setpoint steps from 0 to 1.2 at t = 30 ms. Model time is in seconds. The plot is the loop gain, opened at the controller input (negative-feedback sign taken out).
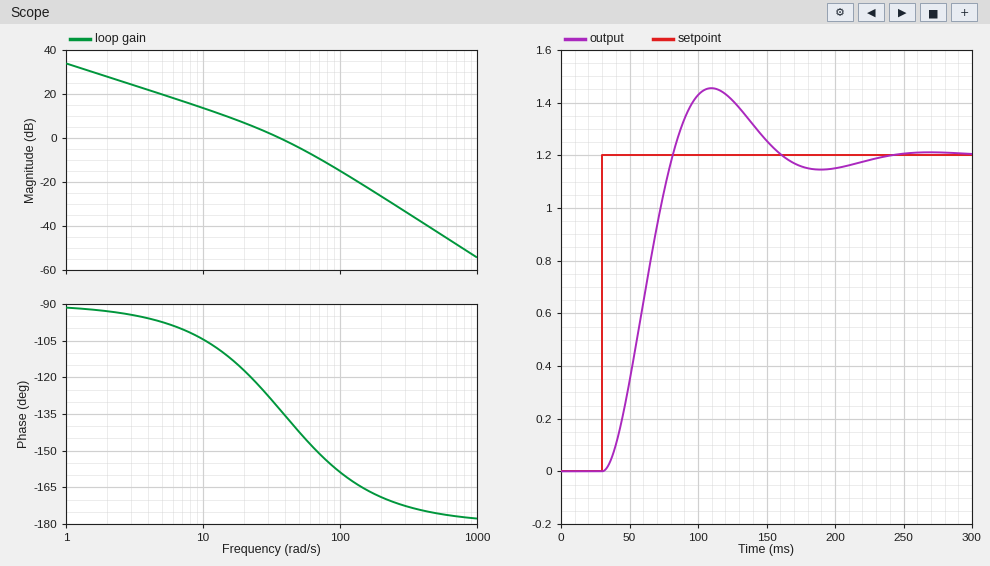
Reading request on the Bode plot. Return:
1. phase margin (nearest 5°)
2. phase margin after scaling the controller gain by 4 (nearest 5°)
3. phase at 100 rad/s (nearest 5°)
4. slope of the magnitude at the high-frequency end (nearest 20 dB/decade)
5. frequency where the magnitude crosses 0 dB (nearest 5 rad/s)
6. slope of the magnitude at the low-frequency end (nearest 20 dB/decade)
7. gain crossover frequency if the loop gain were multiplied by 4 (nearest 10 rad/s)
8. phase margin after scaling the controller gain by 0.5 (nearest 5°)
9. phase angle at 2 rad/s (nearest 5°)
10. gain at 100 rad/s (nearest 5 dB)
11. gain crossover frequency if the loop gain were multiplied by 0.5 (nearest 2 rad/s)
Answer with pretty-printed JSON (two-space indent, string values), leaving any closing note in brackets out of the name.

{
  "phase margin": "45°",
  "phase margin after scaling the controller gain by 4": "25°",
  "phase at 100 rad/s": "-160°",
  "slope of the magnitude at the high-frequency end": "-40 dB/decade",
  "frequency where the magnitude crosses 0 dB": "35 rad/s",
  "slope of the magnitude at the low-frequency end": "-20 dB/decade",
  "gain crossover frequency if the loop gain were multiplied by 4": "80 rad/s",
  "phase margin after scaling the controller gain by 0.5": "60°",
  "phase angle at 2 rad/s": "-95°",
  "gain at 100 rad/s": "-15 dB",
  "gain crossover frequency if the loop gain were multiplied by 0.5": "22 rad/s"
}
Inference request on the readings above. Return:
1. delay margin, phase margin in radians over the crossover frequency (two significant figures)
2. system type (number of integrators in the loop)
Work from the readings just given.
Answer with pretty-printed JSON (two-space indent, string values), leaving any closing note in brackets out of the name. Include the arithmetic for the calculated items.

{
  "delay margin, phase margin in radians over the crossover frequency": "45 × π / 180 / 35 = 0.022 s",
  "system type": "1"
}
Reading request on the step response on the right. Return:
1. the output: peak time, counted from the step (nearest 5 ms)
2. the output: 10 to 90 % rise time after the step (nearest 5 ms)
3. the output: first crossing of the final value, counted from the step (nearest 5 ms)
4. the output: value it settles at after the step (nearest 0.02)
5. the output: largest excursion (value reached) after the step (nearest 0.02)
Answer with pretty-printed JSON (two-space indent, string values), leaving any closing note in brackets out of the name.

{
  "the output: peak time, counted from the step": "80 ms",
  "the output: 10 to 90 % rise time after the step": "35 ms",
  "the output: first crossing of the final value, counted from the step": "50 ms",
  "the output: value it settles at after the step": "1.20",
  "the output: largest excursion (value reached) after the step": "1.46"
}
